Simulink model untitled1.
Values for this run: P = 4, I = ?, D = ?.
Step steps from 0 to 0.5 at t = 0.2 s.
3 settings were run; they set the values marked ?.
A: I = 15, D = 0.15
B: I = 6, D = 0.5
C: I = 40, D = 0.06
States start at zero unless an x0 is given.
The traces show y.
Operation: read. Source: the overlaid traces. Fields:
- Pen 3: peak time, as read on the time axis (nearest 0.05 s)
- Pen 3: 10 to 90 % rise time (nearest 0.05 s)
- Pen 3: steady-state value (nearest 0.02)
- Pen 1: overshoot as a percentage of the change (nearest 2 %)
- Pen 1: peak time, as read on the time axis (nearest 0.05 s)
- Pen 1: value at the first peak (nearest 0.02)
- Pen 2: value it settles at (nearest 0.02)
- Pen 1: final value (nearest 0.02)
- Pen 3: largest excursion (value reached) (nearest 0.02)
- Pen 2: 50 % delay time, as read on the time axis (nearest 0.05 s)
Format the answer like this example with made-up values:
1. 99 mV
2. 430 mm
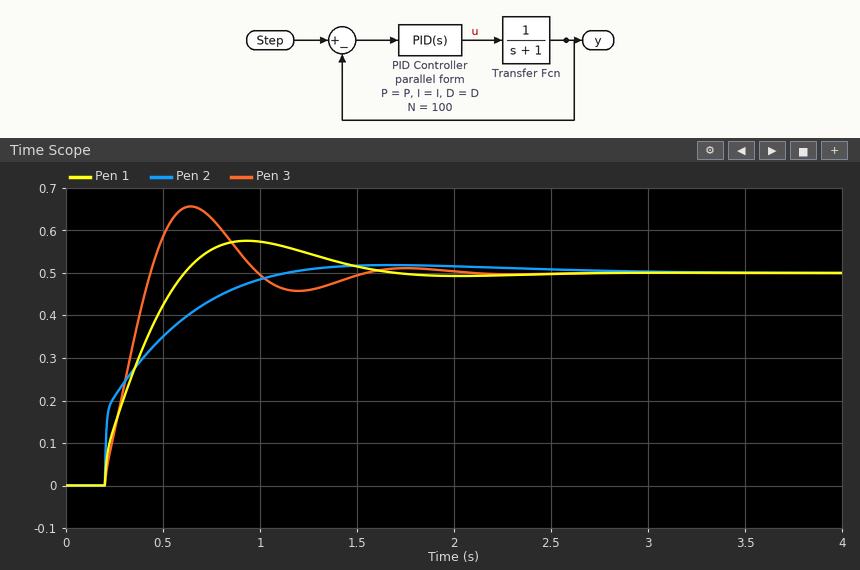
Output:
1. 0.65 s
2. 0.20 s
3. 0.50
4. 16 %
5. 0.95 s
6. 0.58
7. 0.50
8. 0.50
9. 0.66
10. 0.30 s
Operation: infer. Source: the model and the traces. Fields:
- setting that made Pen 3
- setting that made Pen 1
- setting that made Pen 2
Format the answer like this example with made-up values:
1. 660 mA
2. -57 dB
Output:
1. C
2. A
3. B
